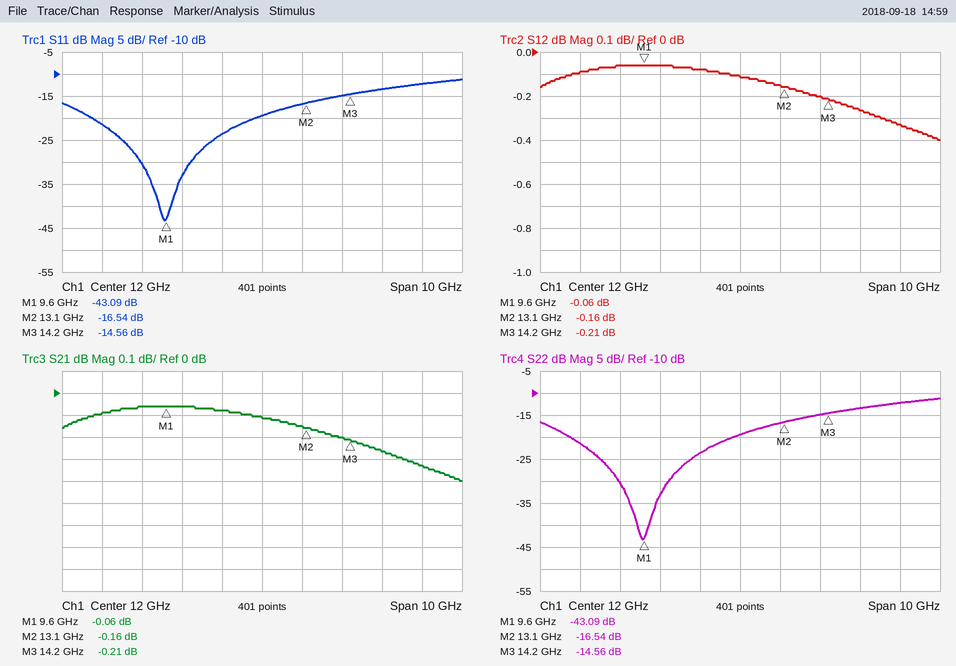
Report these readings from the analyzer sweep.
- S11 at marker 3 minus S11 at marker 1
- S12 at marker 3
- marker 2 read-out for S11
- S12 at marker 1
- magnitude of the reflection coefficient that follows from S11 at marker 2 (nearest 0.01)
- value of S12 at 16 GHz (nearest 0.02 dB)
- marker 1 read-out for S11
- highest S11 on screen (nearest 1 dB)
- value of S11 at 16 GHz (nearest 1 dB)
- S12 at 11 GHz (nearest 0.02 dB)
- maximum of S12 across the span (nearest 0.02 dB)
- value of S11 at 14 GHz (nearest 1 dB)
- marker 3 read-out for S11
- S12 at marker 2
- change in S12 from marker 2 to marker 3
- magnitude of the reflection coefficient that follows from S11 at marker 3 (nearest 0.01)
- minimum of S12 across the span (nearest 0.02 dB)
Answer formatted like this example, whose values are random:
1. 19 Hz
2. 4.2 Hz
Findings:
1. 28.53 dB
2. -0.21 dB
3. -16.54 dB
4. -0.06 dB
5. 0.15
6. -0.32 dB
7. -43.09 dB
8. -11 dB
9. -12 dB
10. -0.08 dB
11. -0.06 dB
12. -15 dB
13. -14.56 dB
14. -0.16 dB
15. -0.05 dB
16. 0.19
17. -0.40 dB
